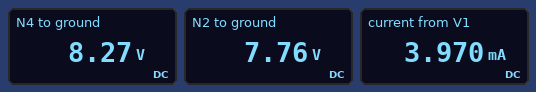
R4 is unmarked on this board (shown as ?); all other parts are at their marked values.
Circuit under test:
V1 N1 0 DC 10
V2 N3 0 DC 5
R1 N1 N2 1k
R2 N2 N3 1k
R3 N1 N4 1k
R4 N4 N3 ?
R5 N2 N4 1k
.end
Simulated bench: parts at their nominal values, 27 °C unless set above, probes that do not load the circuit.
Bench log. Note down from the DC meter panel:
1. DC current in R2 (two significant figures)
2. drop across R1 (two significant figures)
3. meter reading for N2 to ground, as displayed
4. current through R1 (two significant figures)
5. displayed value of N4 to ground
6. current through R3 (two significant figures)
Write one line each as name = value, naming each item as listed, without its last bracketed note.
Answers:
DC current in R2 = 2.8 mA
drop across R1 = 2.2 V
meter reading for N2 to ground, as displayed = 7.76 V
current through R1 = 2.2 mA
displayed value of N4 to ground = 8.27 V
current through R3 = 1.7 mA
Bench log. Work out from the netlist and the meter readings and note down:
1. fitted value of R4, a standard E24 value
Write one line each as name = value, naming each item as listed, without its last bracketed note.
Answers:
fitted value of R4, a standard E24 value = 2.7 kΩ
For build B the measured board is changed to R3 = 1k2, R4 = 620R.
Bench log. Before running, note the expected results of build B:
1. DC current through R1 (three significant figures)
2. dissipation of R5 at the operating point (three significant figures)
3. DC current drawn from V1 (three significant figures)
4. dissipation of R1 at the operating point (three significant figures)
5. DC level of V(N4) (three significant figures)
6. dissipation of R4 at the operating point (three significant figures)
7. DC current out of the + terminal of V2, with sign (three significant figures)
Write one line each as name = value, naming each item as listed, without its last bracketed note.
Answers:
DC current through R1 = 2.71 mA
dissipation of R5 at the operating point = 174 µW
DC current drawn from V1 = 5.31 mA
dissipation of R1 at the operating point = 7.34 mW
DC level of V(N4) = 6.87 V
dissipation of R4 at the operating point = 5.66 mW
DC current out of the + terminal of V2, with sign = -5.31 mA
